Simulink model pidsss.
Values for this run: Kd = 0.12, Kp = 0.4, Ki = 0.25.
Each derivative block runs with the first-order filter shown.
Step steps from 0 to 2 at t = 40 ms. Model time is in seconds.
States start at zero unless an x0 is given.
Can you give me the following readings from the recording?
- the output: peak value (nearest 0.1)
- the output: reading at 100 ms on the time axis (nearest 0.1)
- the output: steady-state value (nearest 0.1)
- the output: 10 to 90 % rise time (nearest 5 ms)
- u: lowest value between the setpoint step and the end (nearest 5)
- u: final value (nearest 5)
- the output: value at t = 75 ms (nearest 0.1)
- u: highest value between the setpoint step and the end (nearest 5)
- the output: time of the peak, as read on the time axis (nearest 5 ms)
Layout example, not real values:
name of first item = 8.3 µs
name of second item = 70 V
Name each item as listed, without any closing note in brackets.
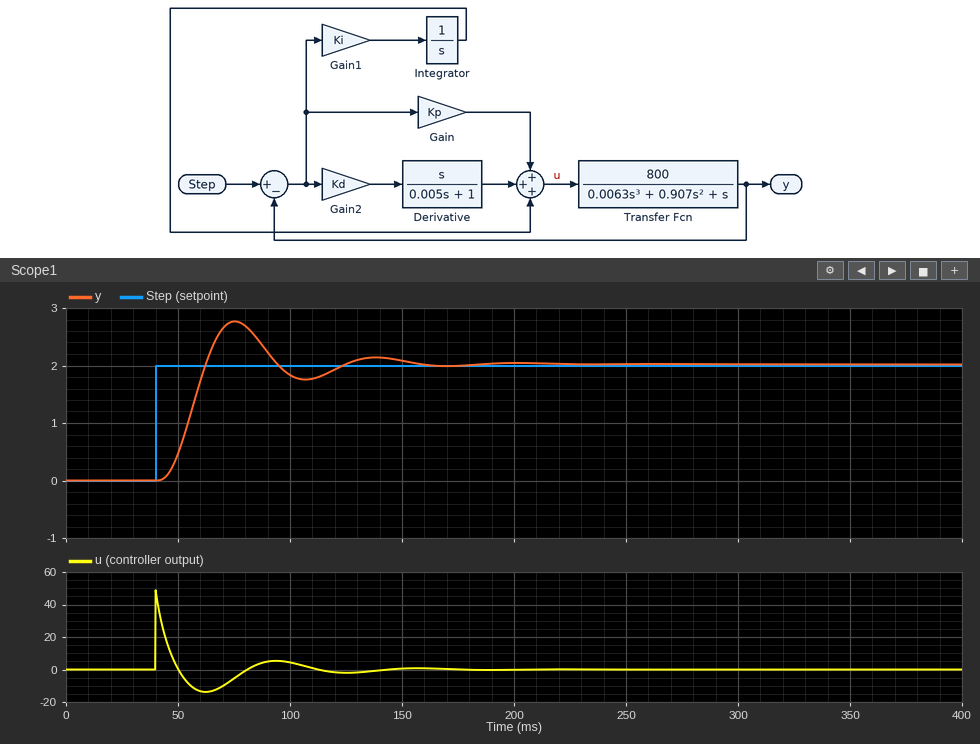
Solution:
the output: peak value = 2.8
the output: reading at 100 ms on the time axis = 1.8
the output: steady-state value = 2.0
the output: 10 to 90 % rise time = 15 ms
u: lowest value between the setpoint step and the end = -15
u: final value = 0
the output: value at t = 75 ms = 2.8
u: highest value between the setpoint step and the end = 50
the output: time of the peak, as read on the time axis = 75 ms
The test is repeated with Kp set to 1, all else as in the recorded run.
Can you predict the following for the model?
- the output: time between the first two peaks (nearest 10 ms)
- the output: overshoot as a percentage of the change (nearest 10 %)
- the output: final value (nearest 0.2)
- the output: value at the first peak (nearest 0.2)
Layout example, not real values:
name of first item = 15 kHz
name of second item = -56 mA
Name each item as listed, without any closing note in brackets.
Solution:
the output: time between the first two peaks = 60 ms
the output: overshoot as a percentage of the change = 50 %
the output: final value = 2.0
the output: value at the first peak = 3.0
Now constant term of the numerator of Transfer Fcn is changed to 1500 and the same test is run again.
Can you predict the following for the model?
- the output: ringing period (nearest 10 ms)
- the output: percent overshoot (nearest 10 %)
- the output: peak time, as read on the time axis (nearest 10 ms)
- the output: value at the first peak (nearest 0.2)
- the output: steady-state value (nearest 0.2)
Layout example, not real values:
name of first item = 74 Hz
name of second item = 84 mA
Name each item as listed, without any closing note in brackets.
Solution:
the output: ringing period = 50 ms
the output: percent overshoot = 70 %
the output: peak time, as read on the time axis = 70 ms
the output: value at the first peak = 3.4
the output: steady-state value = 2.0
